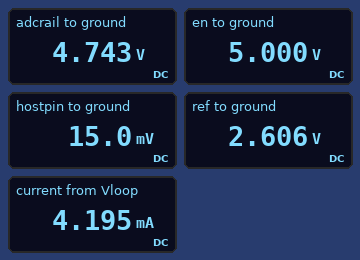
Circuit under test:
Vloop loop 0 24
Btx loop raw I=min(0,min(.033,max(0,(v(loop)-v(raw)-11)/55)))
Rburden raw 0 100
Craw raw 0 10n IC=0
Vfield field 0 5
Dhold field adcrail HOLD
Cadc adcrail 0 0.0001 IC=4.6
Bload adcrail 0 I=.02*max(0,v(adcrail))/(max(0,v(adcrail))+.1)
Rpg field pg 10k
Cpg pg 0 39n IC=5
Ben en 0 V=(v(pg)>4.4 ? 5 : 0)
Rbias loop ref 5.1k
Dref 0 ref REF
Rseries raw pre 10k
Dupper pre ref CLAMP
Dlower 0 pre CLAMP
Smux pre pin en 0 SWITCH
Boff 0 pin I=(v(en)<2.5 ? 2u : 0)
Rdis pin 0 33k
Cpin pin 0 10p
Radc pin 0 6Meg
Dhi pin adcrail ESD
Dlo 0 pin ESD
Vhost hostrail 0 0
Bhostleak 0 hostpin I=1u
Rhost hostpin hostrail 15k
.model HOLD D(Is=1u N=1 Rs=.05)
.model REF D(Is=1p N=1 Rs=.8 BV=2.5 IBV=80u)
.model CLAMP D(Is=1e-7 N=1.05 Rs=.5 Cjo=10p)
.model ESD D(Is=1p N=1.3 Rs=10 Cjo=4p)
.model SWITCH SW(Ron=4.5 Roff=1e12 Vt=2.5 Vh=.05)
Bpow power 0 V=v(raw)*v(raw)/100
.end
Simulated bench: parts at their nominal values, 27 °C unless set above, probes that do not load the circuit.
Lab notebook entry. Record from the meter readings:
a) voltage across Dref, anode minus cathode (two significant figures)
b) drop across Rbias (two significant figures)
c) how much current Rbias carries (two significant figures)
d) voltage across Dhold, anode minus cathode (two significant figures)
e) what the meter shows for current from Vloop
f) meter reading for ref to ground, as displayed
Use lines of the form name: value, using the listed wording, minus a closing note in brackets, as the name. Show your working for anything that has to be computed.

voltage across Dref, anode minus cathode: 0 V - 2.606 V = -2.6 V
drop across Rbias: 24 V - 2.606 V = 21 V
how much current Rbias carries: (24 V - 2.606 V) / 5.1 kΩ = 4.2 mA
voltage across Dhold, anode minus cathode: 5 V - 4.743 V = 260 mV
what the meter shows for current from Vloop: 4.195 mA
meter reading for ref to ground, as displayed: 2.606 V
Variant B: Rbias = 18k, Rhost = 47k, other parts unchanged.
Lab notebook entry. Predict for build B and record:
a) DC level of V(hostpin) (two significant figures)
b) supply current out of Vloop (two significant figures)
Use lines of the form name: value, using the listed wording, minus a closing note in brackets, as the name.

DC level of V(hostpin): 47 mV
supply current out of Vloop: 1.2 mA
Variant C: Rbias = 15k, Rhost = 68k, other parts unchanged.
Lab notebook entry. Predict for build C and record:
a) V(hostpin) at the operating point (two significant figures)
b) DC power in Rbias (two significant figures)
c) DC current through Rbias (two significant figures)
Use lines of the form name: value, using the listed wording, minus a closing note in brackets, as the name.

V(hostpin) at the operating point: 68 mV
DC power in Rbias: 31 mW
DC current through Rbias: 1.4 mA
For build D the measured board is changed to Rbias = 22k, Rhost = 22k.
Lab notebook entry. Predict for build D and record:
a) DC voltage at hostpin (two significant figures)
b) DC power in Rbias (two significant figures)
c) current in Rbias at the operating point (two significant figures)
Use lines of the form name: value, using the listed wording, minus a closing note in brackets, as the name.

DC voltage at hostpin: 22 mV
DC power in Rbias: 21 mW
current in Rbias at the operating point: 970 µA
